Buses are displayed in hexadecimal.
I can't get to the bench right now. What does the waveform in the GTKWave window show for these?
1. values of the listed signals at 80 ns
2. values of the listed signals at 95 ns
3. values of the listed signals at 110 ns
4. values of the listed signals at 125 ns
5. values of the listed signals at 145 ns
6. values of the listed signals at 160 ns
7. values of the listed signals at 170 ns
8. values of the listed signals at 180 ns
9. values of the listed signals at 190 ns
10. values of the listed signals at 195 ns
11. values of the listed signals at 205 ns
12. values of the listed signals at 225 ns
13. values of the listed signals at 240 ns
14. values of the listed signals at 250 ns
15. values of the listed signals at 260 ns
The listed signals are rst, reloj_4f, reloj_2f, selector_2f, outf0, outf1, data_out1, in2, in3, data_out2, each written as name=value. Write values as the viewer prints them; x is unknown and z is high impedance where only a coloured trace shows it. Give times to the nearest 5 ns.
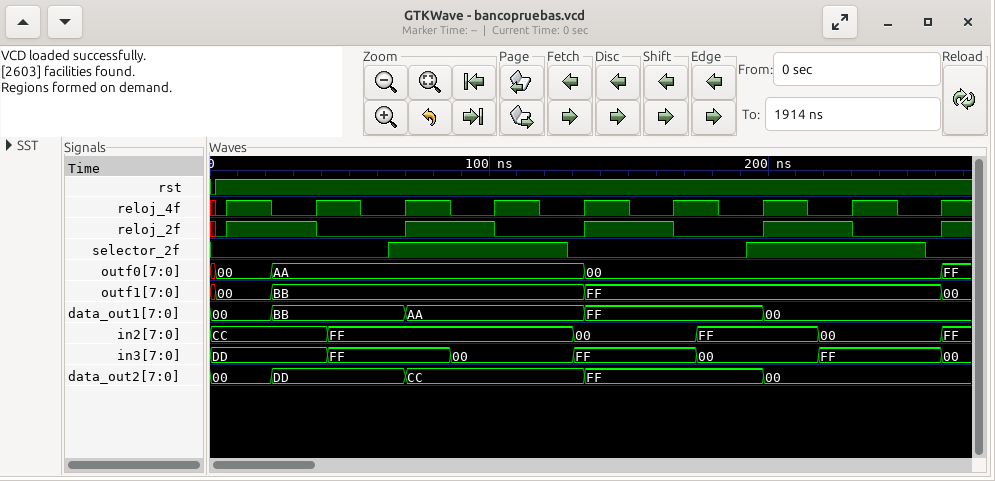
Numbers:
rst=1, reloj_4f=1, reloj_2f=1, selector_2f=1, outf0=AA, outf1=BB, data_out1=AA, in2=FF, in3=FF, data_out2=CC
rst=1, reloj_4f=0, reloj_2f=1, selector_2f=1, outf0=AA, outf1=BB, data_out1=AA, in2=FF, in3=00, data_out2=CC
rst=1, reloj_4f=1, reloj_2f=0, selector_2f=1, outf0=AA, outf1=BB, data_out1=AA, in2=FF, in3=00, data_out2=CC
rst=1, reloj_4f=0, reloj_2f=0, selector_2f=1, outf0=AA, outf1=BB, data_out1=AA, in2=FF, in3=00, data_out2=CC
rst=1, reloj_4f=1, reloj_2f=1, selector_2f=0, outf0=00, outf1=FF, data_out1=FF, in2=00, in3=FF, data_out2=FF
rst=1, reloj_4f=0, reloj_2f=1, selector_2f=0, outf0=00, outf1=FF, data_out1=FF, in2=00, in3=FF, data_out2=FF
rst=1, reloj_4f=1, reloj_2f=0, selector_2f=0, outf0=00, outf1=FF, data_out1=FF, in2=00, in3=FF, data_out2=FF
rst=1, reloj_4f=1, reloj_2f=0, selector_2f=0, outf0=00, outf1=FF, data_out1=FF, in2=FF, in3=00, data_out2=FF
rst=1, reloj_4f=0, reloj_2f=0, selector_2f=0, outf0=00, outf1=FF, data_out1=FF, in2=FF, in3=00, data_out2=FF
rst=1, reloj_4f=0, reloj_2f=0, selector_2f=1, outf0=00, outf1=FF, data_out1=FF, in2=FF, in3=00, data_out2=FF
rst=1, reloj_4f=1, reloj_2f=1, selector_2f=1, outf0=00, outf1=FF, data_out1=00, in2=FF, in3=00, data_out2=00
rst=1, reloj_4f=0, reloj_2f=1, selector_2f=1, outf0=00, outf1=FF, data_out1=00, in2=00, in3=FF, data_out2=00
rst=1, reloj_4f=1, reloj_2f=0, selector_2f=1, outf0=00, outf1=FF, data_out1=00, in2=00, in3=FF, data_out2=00
rst=1, reloj_4f=0, reloj_2f=0, selector_2f=1, outf0=00, outf1=FF, data_out1=00, in2=00, in3=FF, data_out2=00
rst=1, reloj_4f=0, reloj_2f=0, selector_2f=0, outf0=00, outf1=FF, data_out1=00, in2=00, in3=FF, data_out2=00
